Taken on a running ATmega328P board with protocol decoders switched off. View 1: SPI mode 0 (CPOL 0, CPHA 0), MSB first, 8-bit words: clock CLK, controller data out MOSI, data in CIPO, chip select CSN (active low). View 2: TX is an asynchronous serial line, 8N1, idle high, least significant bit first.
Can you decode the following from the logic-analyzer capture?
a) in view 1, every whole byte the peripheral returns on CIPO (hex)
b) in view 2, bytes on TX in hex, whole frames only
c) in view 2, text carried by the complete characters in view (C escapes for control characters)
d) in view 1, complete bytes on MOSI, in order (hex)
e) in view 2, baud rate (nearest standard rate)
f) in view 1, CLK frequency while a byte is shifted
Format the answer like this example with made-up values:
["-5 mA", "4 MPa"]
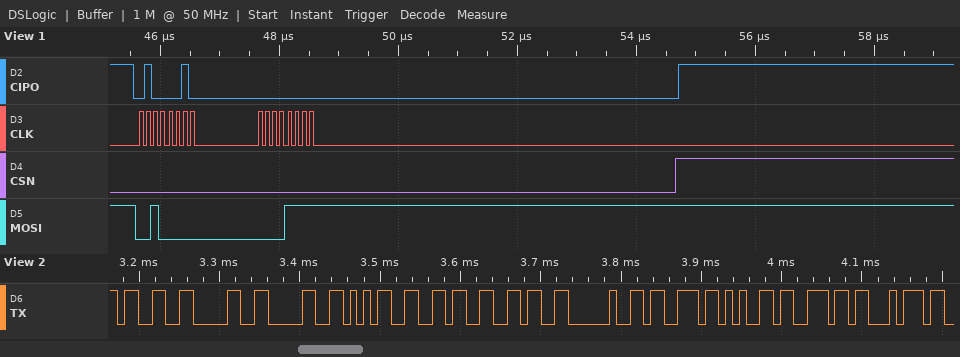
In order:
["42 00", "33 30 30 35 36 36 20 73 65 6E 74", "\"300566 sent\"", "20 0F", "115200 baud", "8 MHz"]
